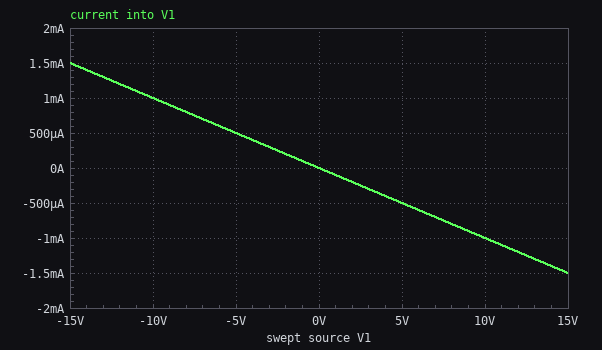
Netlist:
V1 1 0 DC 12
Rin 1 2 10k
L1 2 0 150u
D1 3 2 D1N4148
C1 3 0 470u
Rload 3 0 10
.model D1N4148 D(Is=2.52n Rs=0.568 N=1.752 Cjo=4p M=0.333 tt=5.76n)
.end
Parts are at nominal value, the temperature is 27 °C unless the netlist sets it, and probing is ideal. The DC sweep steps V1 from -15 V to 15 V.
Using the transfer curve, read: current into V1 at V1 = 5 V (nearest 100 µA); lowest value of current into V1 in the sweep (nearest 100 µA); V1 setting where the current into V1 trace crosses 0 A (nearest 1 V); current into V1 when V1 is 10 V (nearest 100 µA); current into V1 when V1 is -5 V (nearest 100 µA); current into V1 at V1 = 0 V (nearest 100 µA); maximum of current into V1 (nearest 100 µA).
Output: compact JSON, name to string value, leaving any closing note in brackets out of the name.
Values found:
{"current into V1 at V1 = 5 V": "-500 µA", "lowest value of current into V1 in the sweep": "-1.5 mA", "V1 setting where the current into V1 trace crosses 0 A": "0 V", "current into V1 when V1 is 10 V": "-1.0 mA", "current into V1 when V1 is -5 V": "500 µA", "current into V1 at V1 = 0 V": "0 A", "maximum of current into V1": "1.5 mA"}
